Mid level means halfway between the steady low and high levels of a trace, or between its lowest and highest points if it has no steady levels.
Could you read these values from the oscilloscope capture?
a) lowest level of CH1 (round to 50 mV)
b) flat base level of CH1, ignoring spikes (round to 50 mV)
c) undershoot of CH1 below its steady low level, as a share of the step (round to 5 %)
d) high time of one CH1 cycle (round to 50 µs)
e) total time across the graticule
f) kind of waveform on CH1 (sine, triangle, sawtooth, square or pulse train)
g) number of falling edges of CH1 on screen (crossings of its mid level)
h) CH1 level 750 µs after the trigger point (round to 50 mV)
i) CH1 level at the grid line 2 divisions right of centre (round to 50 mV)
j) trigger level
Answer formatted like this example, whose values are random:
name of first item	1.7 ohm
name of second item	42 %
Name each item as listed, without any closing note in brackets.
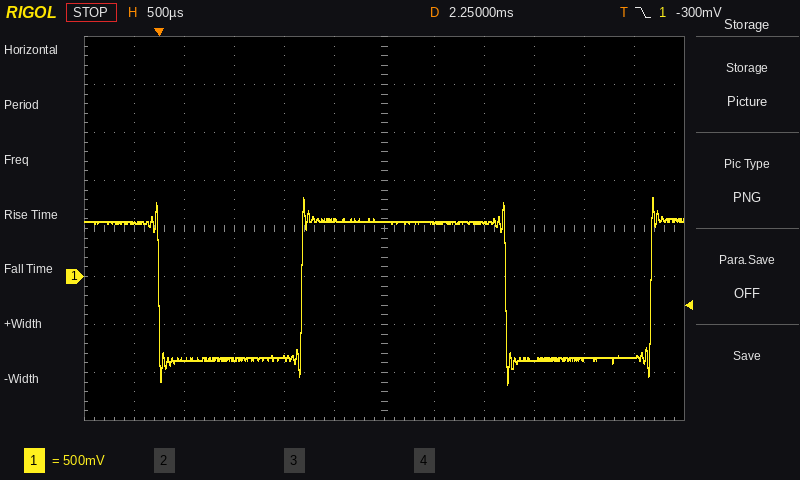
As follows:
lowest level of CH1	-1.10 V
flat base level of CH1, ignoring spikes	-850 mV
undershoot of CH1 below its steady low level, as a share of the step	20 %
high time of one CH1 cycle	2.05 ms
total time across the graticule	6 ms
kind of waveform on CH1	pulse train
number of falling edges of CH1 on screen	2
CH1 level 750 µs after the trigger point	-850 mV
CH1 level at the grid line 2 divisions right of centre	550 mV
trigger level	-300 mV
